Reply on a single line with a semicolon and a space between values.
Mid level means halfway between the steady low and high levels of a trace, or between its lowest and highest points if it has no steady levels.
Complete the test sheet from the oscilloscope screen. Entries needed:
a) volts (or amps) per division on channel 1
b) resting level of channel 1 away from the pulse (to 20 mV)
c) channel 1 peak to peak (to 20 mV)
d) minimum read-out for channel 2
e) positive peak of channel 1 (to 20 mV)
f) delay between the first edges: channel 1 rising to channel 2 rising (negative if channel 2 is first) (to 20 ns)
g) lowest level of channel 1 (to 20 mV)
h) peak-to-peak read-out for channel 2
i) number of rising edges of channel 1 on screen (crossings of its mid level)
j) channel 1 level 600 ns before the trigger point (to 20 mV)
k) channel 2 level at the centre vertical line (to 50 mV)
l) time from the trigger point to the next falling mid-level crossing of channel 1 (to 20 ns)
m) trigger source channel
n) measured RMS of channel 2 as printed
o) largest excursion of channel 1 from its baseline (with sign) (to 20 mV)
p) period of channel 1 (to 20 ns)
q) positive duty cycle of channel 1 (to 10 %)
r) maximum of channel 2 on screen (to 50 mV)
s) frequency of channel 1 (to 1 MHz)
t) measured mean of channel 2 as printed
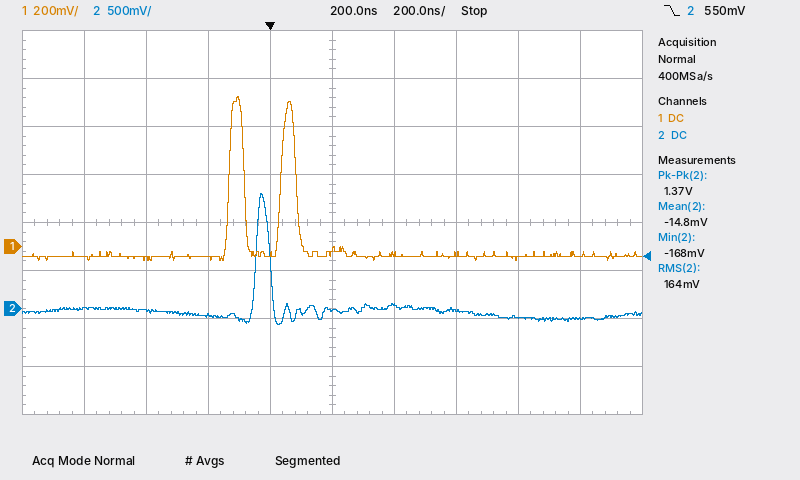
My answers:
200 mV; -40 mV; 680 mV; -168 mV; 620 mV; +80 ns; -60 mV; 1.37 V; 2; -40 mV; 0 mV; 80 ns; channel 2; 164 mV; +660 mV; 160 ns; 30 %; 1.20 V; 6 MHz; -14.8 mV
